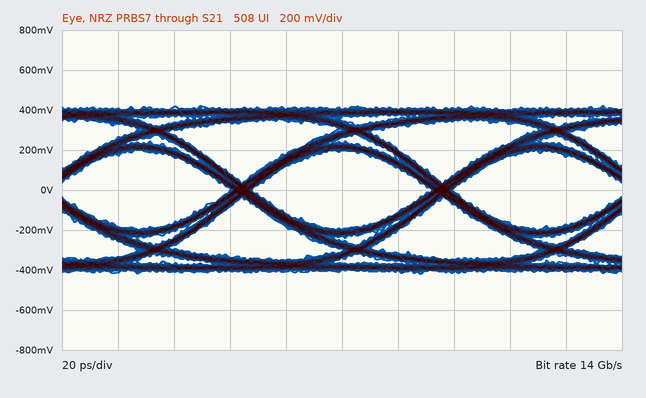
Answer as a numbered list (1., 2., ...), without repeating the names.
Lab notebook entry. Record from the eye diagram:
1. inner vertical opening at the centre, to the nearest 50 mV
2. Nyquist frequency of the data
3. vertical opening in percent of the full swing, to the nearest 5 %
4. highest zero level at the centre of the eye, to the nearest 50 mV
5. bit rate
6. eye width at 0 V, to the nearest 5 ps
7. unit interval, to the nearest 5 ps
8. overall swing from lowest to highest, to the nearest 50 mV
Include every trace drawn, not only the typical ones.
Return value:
1. 400 mV
2. 7 GHz
3. 45 %
4. -200 mV
5. 14 Gb/s
6. 65 ps
7. 70 ps
8. 850 mV
